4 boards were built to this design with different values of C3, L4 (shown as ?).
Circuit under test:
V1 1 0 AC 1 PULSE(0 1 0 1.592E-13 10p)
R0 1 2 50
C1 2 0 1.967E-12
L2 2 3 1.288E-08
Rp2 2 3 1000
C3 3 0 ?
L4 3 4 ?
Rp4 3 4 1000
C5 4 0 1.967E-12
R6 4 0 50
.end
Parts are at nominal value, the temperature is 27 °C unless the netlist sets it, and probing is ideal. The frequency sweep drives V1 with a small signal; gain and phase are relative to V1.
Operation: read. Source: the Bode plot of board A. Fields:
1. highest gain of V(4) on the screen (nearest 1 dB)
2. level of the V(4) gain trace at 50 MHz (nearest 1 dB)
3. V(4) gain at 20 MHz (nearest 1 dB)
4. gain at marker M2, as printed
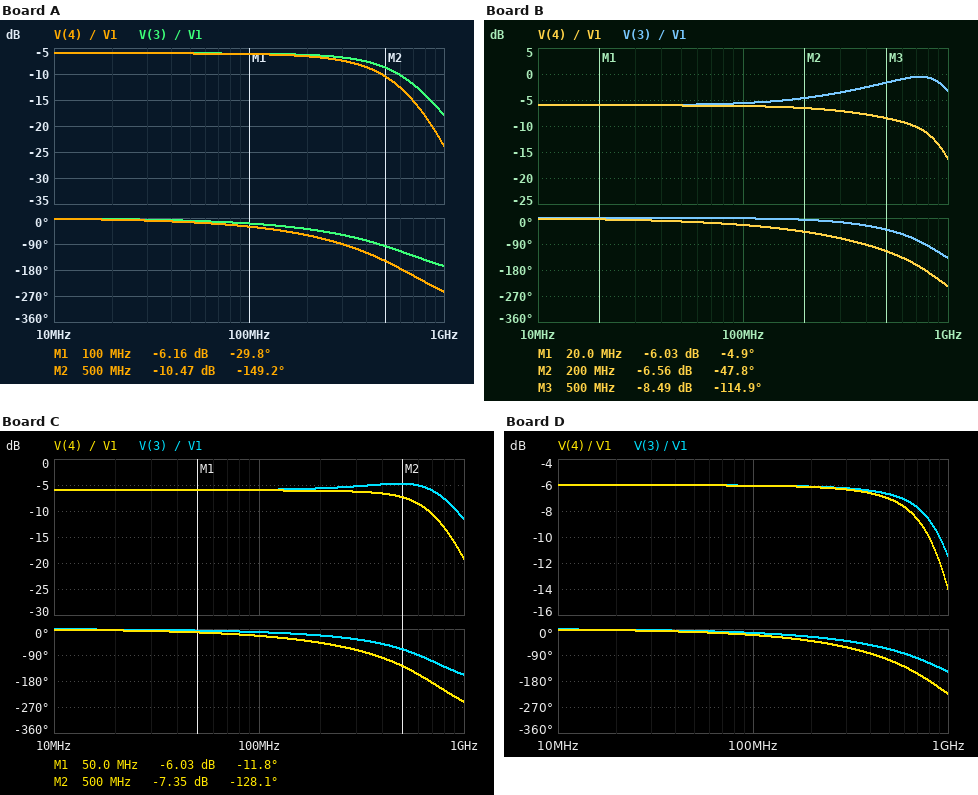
-6 dB
-6 dB
-6 dB
-10.47 dB
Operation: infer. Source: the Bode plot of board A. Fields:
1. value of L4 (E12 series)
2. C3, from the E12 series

15 nH
18 pF
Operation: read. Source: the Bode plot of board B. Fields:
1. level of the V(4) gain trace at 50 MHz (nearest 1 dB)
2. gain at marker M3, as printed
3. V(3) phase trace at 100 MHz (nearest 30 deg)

-6 dB
-8.49 dB
0 deg
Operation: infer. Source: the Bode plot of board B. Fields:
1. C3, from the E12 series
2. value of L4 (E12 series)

4.7 pF
33 nH
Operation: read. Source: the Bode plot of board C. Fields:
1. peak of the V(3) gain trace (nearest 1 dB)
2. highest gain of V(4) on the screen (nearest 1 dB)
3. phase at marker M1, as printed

-5 dB
-6 dB
-11.8 deg
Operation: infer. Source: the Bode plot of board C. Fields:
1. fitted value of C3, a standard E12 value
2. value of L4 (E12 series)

10 pF
18 nH
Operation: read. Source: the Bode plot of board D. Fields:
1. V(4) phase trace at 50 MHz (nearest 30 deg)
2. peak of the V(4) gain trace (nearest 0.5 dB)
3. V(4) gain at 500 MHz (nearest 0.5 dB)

0 deg
-6.0 dB
-7.0 dB
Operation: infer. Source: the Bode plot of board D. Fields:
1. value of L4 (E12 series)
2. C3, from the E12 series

10 nH
10 pF
